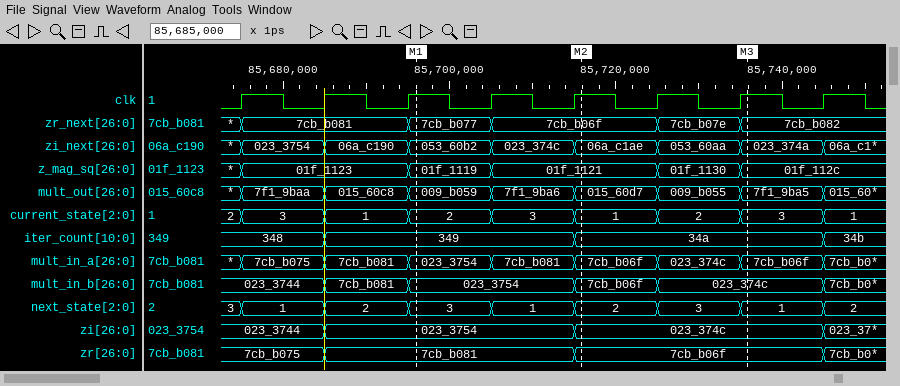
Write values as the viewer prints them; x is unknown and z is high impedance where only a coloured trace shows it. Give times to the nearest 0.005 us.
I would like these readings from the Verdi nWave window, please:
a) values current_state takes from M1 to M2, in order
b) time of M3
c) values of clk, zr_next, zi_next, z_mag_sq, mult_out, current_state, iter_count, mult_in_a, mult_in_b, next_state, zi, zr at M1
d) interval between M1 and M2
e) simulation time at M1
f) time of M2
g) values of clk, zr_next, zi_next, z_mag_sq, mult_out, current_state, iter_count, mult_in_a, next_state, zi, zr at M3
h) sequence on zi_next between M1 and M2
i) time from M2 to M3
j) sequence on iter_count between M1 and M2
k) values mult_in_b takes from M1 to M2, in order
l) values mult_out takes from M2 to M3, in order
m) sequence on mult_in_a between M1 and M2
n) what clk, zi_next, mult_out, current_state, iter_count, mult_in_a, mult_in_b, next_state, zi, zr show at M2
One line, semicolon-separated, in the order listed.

2, 3, 1; 85.735 us; clk=1, zr_next=7cb_b077, zi_next=053_60b2, z_mag_sq=01f_1119, mult_out=009_b059, current_state=2, iter_count=349, mult_in_a=023_3754, mult_in_b=023_3754, next_state=3, zi=023_3754, zr=7cb_b081; 0.02 us; 85.695 us; 85.715 us; clk=1, zr_next=7cb_b082, zi_next=023_374a, z_mag_sq=01f_112c, mult_out=7f1_9ba5, current_state=3, iter_count=34a, mult_in_a=7cb_b06f, next_state=1, zi=023_374c, zr=7cb_b06f; 053_60b2, 023_374c, 06a_c1ae; 0.02 us; 349, 34a; 023_3754, 7cb_b06f; 015_60d7, 009_b055, 7f1_9ba5; 023_3754, 7cb_b081, 7cb_b06f; clk=1, zi_next=06a_c1ae, mult_out=015_60d7, current_state=1, iter_count=34a, mult_in_a=7cb_b06f, mult_in_b=7cb_b06f, next_state=2, zi=023_374c, zr=7cb_b06f
